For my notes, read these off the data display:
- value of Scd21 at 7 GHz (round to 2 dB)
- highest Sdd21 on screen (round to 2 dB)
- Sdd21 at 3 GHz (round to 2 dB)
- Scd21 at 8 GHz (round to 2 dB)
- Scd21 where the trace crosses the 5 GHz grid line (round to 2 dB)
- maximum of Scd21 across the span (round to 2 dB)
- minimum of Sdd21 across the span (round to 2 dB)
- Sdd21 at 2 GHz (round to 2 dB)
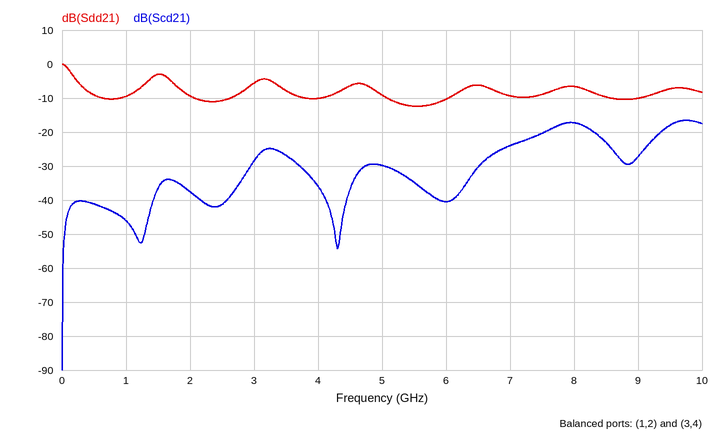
-24 dB
0 dB
-6 dB
-18 dB
-30 dB
-16 dB
-12 dB
-10 dB
